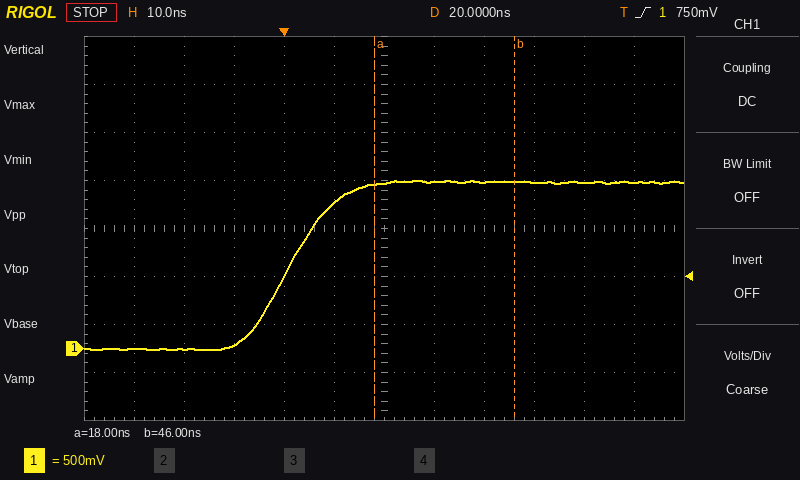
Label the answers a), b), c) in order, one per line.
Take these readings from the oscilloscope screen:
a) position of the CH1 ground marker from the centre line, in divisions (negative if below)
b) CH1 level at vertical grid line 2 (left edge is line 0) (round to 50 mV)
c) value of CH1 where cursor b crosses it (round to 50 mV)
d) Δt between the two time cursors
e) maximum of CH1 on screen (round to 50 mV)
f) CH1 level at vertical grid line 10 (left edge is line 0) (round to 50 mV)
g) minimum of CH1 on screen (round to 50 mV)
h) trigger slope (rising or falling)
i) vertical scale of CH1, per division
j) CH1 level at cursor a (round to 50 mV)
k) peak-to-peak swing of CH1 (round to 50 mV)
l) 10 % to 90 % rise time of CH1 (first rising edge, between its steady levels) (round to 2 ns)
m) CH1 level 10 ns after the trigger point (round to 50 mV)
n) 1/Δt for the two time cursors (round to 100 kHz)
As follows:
a) -2.5 div
b) 0 mV
c) 1.75 V
d) 28 ns
e) 1.75 V
f) 1.75 V
g) 0 mV
h) rising
i) 500 mV
j) 1.70 V
k) 1.75 V
l) 18 ns
m) 1.50 V
n) 35.7 MHz
